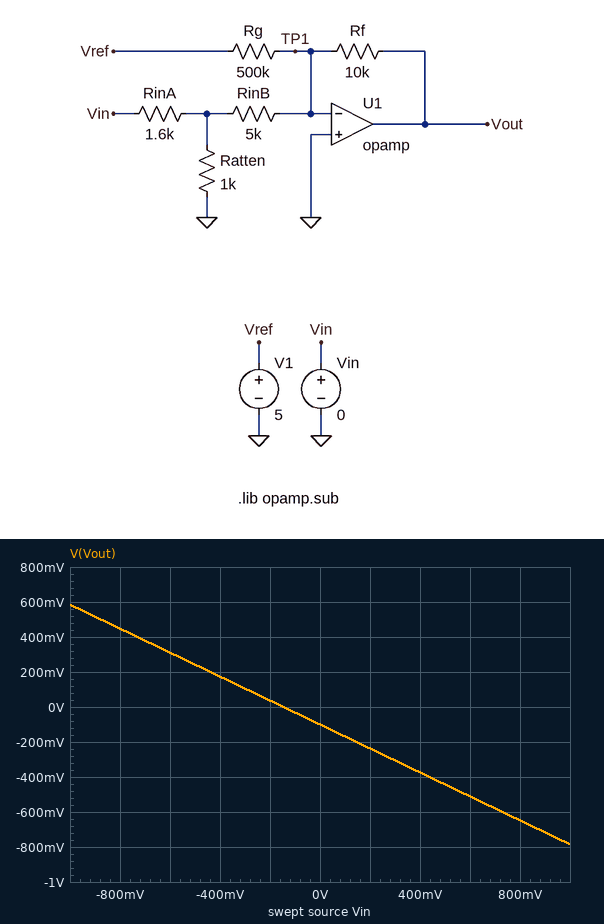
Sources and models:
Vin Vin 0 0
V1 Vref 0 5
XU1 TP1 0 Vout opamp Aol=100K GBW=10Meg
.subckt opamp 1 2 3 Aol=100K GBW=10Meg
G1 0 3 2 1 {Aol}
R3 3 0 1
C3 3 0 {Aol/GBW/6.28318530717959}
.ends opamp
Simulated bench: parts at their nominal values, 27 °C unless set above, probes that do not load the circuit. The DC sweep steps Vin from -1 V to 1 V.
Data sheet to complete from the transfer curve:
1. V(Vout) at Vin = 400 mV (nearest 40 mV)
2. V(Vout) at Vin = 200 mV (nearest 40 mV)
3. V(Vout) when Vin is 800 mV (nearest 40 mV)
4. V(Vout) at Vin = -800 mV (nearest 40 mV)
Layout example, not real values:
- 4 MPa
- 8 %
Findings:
- -360 mV
- -240 mV
- -640 mV
- 440 mV
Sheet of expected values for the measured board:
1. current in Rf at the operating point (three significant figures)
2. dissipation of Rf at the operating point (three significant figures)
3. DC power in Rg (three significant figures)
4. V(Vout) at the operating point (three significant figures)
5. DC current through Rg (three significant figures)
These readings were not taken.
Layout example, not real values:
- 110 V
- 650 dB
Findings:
- 10.0 µA
- 1.00 µW
- 50.0 µW
- -100 mV
- 10.0 µA
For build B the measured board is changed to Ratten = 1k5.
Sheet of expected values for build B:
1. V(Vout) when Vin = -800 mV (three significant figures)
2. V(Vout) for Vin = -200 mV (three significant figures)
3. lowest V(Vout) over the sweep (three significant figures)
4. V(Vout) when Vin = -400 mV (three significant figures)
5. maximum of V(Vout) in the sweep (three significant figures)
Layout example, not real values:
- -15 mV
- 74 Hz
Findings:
- 570 mV
- 67.6 mV
- -938 mV
- 235 mV
- 738 mV
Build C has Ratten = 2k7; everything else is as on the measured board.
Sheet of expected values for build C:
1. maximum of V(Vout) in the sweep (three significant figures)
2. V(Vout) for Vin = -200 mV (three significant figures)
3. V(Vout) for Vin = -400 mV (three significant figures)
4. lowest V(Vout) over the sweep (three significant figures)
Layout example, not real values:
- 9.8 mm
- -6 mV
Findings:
- 946 mV
- 109 mV
- 318 mV
- -1.15 V
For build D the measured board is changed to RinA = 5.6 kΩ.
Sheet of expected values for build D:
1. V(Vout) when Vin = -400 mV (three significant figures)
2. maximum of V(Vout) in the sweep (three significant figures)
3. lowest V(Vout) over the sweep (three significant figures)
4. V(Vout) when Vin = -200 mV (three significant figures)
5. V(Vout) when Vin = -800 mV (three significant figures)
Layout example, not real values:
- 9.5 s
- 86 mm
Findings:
- 3.63 mV
- 159 mV
- -359 mV
- -48.2 mV
- 107 mV
